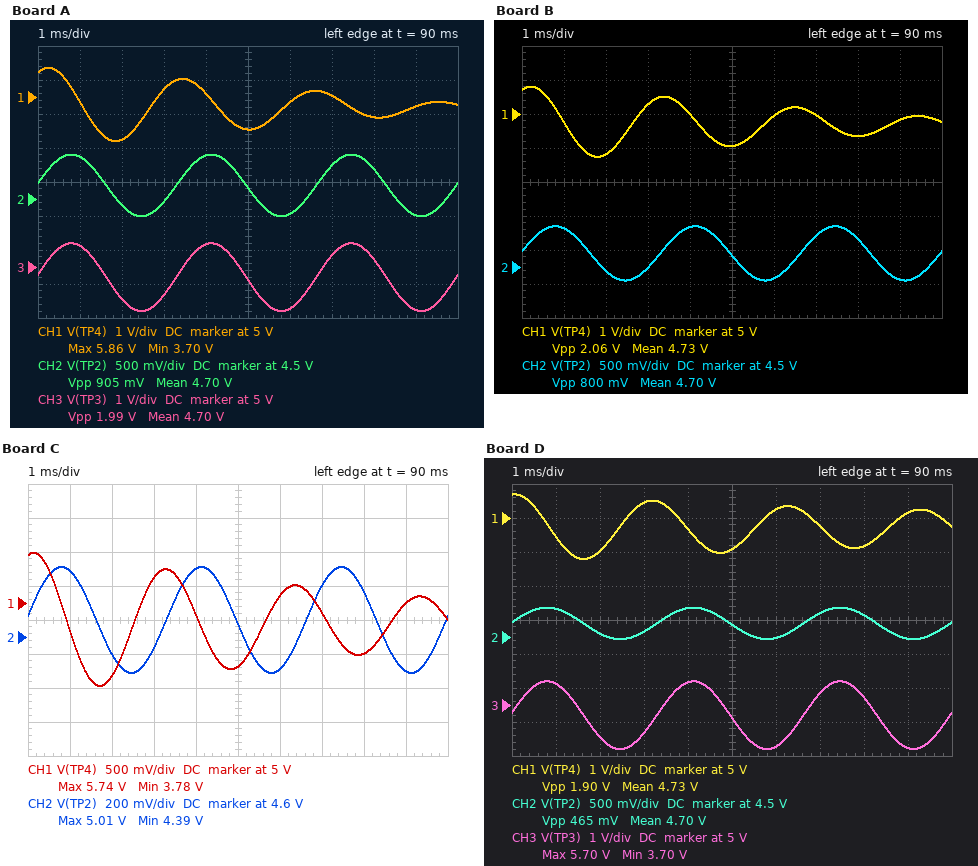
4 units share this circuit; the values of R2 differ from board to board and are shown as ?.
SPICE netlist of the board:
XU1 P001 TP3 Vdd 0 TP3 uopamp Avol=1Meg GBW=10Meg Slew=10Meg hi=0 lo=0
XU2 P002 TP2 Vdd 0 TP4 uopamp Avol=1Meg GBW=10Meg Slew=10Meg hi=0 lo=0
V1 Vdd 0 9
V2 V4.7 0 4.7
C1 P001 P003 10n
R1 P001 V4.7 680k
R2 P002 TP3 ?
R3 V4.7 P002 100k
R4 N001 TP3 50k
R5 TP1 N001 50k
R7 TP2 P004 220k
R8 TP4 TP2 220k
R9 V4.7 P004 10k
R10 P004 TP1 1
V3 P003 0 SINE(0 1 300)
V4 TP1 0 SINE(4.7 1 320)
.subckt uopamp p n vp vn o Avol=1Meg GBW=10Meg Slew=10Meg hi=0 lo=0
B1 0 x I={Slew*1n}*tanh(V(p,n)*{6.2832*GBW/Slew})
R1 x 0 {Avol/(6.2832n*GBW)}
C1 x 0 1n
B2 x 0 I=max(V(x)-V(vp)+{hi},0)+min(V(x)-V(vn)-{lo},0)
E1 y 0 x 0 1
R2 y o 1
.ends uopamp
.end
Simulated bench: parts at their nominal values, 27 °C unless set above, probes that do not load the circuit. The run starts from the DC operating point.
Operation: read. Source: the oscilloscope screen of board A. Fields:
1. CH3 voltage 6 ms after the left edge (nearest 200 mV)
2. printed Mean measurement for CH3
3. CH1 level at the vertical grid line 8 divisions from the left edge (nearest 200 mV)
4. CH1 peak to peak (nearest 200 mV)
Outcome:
3.8 V
4.70 V
4.4 V
2.2 V
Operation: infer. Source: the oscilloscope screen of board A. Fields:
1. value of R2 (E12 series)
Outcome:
120 kΩ
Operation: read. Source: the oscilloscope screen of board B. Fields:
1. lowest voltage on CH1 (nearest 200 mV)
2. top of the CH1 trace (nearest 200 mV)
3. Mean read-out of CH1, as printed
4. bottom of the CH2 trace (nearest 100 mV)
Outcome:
3.8 V
5.8 V
4.73 V
4.3 V
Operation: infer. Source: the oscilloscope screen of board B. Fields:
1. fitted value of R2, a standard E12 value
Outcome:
150 kΩ
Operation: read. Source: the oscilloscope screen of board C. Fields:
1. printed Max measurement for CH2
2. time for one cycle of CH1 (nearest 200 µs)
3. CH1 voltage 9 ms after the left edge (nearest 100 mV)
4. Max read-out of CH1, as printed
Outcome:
5.01 V
3.0 ms
5.0 V
5.74 V
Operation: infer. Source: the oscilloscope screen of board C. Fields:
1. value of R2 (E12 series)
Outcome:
220 kΩ
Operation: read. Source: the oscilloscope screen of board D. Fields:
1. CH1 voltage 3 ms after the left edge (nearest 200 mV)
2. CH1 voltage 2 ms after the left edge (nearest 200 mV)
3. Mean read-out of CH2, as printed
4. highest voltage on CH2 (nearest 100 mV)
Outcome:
5.4 V
4.0 V
4.70 V
4.9 V
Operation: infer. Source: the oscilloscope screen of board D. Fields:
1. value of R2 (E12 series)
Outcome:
330 kΩ
